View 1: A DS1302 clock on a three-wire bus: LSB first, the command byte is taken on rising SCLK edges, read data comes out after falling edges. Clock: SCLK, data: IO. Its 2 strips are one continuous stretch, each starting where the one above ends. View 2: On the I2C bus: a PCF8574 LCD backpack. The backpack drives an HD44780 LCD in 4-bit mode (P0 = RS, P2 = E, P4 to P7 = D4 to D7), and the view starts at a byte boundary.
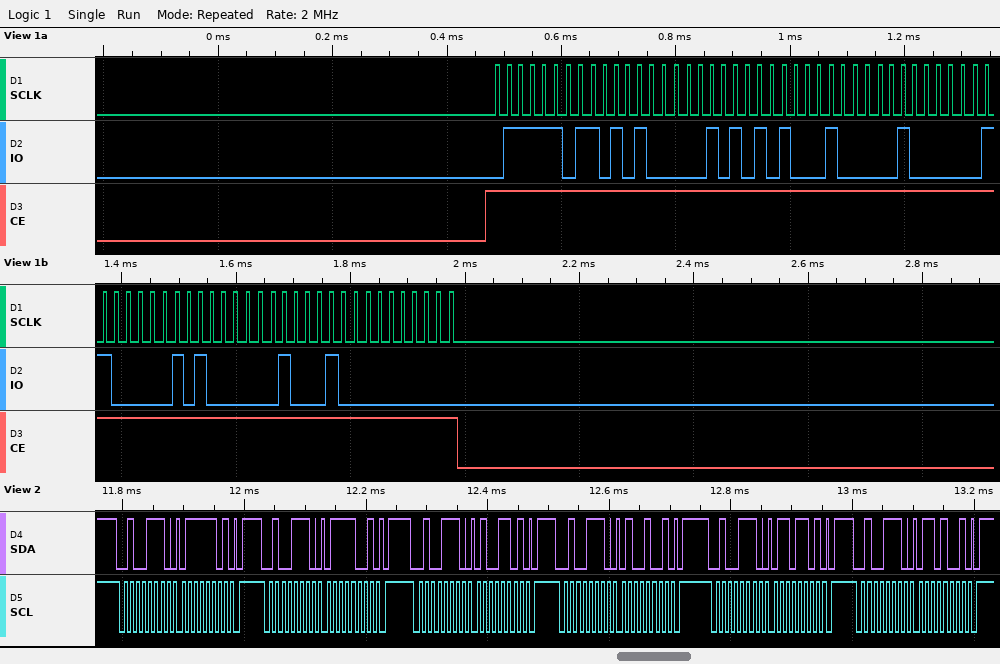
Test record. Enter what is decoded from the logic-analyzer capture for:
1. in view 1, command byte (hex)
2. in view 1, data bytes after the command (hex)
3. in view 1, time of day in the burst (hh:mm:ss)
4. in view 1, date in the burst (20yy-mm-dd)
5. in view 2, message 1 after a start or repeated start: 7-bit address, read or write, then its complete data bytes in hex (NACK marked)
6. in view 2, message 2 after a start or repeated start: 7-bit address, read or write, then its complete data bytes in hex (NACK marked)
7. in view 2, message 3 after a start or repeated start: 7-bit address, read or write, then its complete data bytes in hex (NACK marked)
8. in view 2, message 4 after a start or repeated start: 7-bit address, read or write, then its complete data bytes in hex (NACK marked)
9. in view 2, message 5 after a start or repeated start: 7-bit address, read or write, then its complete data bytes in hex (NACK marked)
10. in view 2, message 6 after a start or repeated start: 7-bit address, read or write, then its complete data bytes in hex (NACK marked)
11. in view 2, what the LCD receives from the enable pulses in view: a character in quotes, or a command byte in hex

0xBE
15 54 11 04 06 05 22 00
11:54:15
2022-06-04
0x27 write: 7D
0x27 write: 79
0x27 write: 4D
0x27 write: 49
0x27 write: 6D
0x27 write: 69
't'
